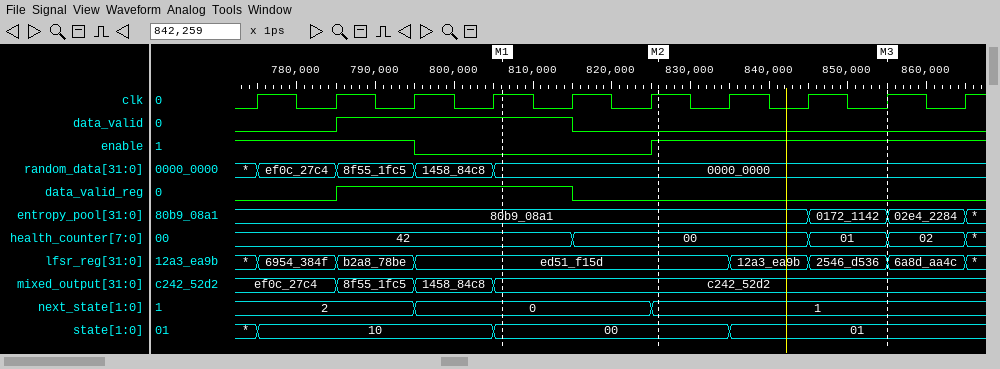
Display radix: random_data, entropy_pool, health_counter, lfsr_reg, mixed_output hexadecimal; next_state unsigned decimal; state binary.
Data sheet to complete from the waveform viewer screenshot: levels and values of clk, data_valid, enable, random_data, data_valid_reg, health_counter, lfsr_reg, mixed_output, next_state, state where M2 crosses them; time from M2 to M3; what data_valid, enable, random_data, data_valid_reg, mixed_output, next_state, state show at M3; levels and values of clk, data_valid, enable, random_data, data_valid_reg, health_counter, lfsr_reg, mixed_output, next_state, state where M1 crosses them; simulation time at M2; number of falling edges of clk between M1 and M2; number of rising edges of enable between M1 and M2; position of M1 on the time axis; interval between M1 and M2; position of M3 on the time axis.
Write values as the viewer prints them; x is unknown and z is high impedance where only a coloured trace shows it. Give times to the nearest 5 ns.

clk=1, data_valid=0, enable=1, random_data=0000_0000, data_valid_reg=0, health_counter=00, lfsr_reg=ed51_f15d, mixed_output=c242_52d2, next_state=1, state=00
30 ns
data_valid=0, enable=1, random_data=0000_0000, data_valid_reg=0, mixed_output=c242_52d2, next_state=1, state=01
clk=1, data_valid=1, enable=0, random_data=0000_0000, data_valid_reg=1, health_counter=42, lfsr_reg=ed51_f15d, mixed_output=c242_52d2, next_state=0, state=00
825 ns
2
1
805 ns
20 ns
855 ns
